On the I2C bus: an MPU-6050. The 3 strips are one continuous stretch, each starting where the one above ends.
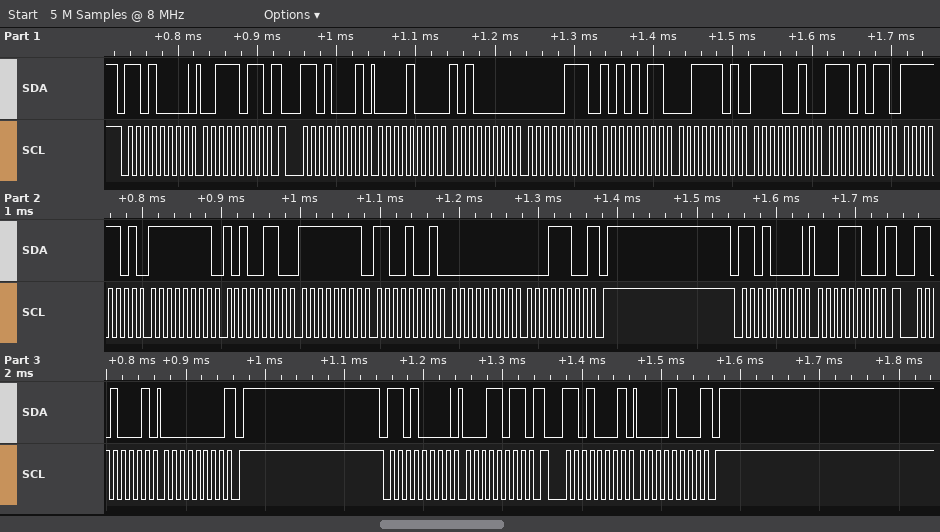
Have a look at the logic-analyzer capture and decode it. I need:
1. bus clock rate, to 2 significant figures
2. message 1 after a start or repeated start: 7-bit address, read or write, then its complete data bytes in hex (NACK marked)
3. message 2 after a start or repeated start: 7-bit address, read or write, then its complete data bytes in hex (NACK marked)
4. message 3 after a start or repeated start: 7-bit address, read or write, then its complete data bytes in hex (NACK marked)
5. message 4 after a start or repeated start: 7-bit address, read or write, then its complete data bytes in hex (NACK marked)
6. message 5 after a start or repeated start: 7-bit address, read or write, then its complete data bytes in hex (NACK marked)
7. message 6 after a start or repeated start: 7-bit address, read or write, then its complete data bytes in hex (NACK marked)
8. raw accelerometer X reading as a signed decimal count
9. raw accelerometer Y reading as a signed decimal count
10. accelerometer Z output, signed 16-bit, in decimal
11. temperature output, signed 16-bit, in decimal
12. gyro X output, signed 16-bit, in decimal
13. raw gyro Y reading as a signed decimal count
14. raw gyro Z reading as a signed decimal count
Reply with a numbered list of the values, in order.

1. 100 kHz
2. 0x68 write: 3B
3. 0x68 read: 08 A0 07 AB 3D F2 EB FD FF A6 FF C9 00 1C NACK
4. 0x68 write: 1C
5. 0x68 read: 00 NACK
6. 0x68 write: 1B
7. 0x68 read: 08 NACK
8. 2208
9. 1963
10. 15858
11. -5123
12. -90
13. -55
14. 28
